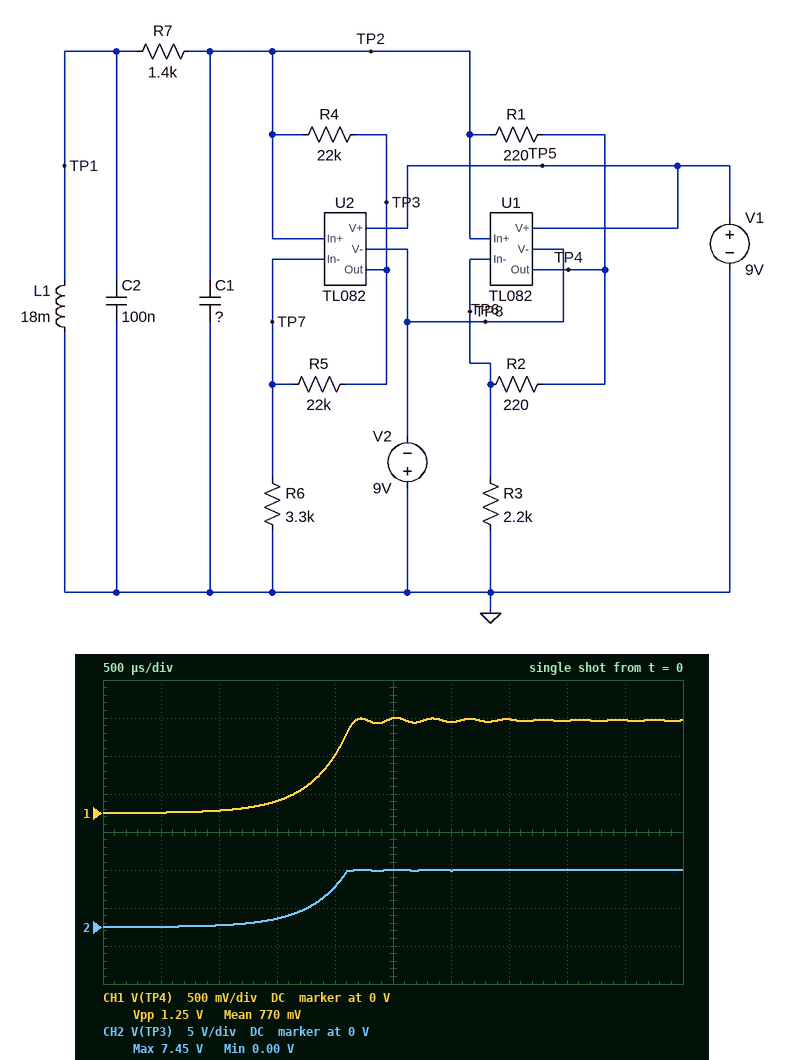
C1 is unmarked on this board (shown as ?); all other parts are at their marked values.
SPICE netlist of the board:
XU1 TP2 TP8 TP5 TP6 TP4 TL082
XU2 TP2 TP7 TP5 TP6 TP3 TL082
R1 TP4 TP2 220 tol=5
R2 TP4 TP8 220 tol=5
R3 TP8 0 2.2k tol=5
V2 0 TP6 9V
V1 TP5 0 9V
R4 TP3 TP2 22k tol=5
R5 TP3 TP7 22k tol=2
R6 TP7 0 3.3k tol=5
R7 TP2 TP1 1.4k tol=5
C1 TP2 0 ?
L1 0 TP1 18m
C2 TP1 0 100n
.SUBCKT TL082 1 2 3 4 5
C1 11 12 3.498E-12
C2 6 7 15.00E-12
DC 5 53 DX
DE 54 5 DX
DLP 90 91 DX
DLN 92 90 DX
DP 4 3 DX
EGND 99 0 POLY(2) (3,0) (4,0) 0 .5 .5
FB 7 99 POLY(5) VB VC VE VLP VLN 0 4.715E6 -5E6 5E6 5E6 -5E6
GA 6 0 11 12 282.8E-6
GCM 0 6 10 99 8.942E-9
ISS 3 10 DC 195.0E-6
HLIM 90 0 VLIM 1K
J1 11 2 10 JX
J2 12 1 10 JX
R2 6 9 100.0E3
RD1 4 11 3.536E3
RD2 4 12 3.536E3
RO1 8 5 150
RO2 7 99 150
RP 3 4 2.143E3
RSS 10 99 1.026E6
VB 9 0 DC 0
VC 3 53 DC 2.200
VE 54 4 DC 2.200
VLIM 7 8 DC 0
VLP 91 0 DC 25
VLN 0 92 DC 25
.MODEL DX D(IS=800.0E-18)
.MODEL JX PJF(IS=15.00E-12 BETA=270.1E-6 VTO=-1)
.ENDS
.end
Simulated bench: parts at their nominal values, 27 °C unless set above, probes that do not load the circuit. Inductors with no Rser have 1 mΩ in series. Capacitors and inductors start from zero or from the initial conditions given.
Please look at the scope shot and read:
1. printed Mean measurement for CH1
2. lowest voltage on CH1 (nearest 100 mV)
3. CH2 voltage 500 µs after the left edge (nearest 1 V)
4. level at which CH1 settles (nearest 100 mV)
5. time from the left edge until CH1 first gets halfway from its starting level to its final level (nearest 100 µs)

770 mV
0 V
0 V
1.2 V
1.9 ms
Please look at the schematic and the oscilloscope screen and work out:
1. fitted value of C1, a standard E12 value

22 nF
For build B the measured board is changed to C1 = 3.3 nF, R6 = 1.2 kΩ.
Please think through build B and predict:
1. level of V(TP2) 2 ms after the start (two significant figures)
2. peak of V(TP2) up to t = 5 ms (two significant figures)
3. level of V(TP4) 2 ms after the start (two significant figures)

-7.7 V
7.7 V
-7.5 V
